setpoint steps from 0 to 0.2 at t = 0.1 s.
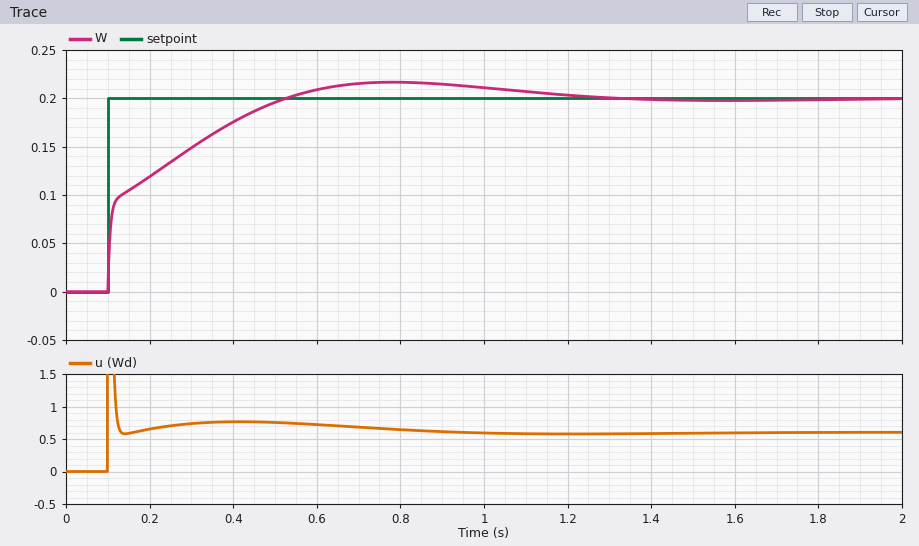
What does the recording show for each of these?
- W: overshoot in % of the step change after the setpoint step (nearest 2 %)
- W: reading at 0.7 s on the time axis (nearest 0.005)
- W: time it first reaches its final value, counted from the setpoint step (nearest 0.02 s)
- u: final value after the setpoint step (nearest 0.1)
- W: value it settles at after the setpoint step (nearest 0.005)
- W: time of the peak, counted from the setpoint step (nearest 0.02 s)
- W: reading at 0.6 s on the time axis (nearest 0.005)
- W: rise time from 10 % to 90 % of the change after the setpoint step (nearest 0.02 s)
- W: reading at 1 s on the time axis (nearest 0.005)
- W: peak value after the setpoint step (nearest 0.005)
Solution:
8 %
0.215
0.42 s
0.6
0.200
0.68 s
0.210
0.32 s
0.210
0.215
